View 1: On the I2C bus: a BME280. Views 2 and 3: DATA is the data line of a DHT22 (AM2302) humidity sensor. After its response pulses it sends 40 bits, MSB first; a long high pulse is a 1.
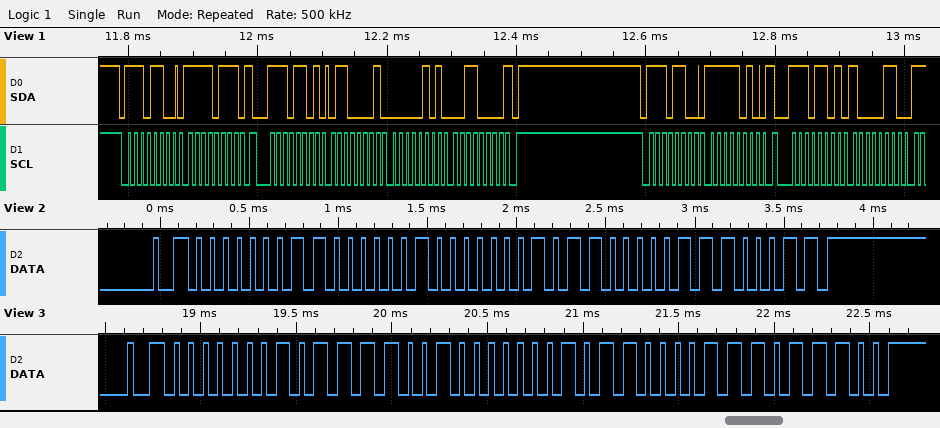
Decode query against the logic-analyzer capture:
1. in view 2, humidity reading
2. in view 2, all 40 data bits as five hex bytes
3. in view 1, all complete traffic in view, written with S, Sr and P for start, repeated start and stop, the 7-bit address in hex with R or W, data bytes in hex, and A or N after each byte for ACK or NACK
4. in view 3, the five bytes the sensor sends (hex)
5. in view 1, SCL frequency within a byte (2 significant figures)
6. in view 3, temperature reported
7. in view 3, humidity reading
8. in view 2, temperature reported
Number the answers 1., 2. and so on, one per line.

1. 38.5 %
2. 01 81 01 60 E3
3. S 76W A F7 A Sr 76R A 61 A 05 A 30 N P S 76W A FA A Sr 76R A 86 A
4. 01 79 01 61 DC
5. 100 kHz
6. 35.3 °C
7. 37.7 %
8. 35.2 °C
